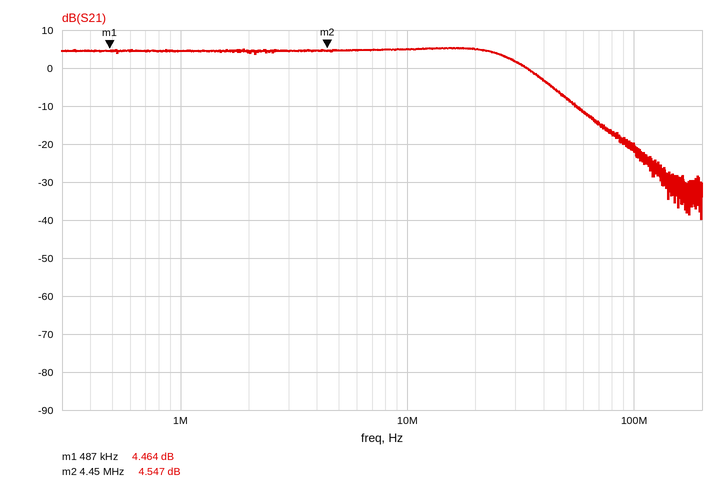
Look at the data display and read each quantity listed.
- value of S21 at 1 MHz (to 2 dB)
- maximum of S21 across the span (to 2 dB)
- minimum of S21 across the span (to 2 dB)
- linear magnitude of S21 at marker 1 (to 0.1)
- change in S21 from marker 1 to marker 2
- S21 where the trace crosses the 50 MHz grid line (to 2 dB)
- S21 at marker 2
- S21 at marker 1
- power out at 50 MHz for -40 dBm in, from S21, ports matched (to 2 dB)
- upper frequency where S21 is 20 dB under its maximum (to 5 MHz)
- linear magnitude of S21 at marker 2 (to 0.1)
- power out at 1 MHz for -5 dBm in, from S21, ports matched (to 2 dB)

4 dB
6 dB
-40 dB
1.7
0.083 dB
-8 dB
4.547 dB
4.464 dB
-48 dBm
70 MHz
1.7
0 dBm
